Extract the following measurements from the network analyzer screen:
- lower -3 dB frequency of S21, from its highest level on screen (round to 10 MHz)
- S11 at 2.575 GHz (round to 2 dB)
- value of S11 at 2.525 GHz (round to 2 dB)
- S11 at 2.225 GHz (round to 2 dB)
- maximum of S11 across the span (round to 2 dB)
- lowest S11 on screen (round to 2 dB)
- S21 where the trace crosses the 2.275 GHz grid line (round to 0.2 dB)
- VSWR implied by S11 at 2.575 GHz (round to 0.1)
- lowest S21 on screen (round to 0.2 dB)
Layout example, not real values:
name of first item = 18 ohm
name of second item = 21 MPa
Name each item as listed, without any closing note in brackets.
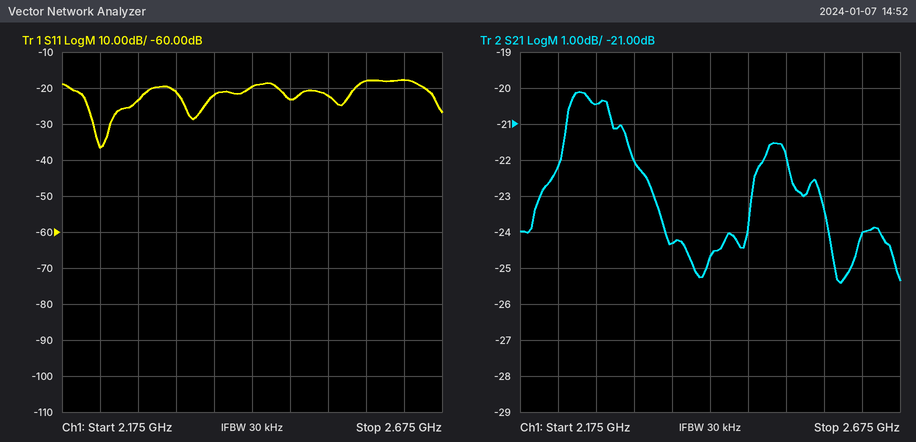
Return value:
lower -3 dB frequency of S21, from its highest level on screen = 2.20 GHz
S11 at 2.575 GHz = -18 dB
value of S11 at 2.525 GHz = -22 dB
S11 at 2.225 GHz = -36 dB
maximum of S11 across the span = -18 dB
lowest S11 on screen = -36 dB
S21 where the trace crosses the 2.275 GHz grid line = -20.4 dB
VSWR implied by S11 at 2.575 GHz = 1.3
lowest S21 on screen = -25.4 dB
